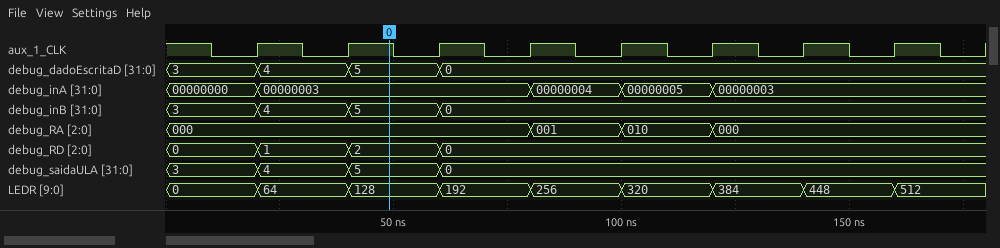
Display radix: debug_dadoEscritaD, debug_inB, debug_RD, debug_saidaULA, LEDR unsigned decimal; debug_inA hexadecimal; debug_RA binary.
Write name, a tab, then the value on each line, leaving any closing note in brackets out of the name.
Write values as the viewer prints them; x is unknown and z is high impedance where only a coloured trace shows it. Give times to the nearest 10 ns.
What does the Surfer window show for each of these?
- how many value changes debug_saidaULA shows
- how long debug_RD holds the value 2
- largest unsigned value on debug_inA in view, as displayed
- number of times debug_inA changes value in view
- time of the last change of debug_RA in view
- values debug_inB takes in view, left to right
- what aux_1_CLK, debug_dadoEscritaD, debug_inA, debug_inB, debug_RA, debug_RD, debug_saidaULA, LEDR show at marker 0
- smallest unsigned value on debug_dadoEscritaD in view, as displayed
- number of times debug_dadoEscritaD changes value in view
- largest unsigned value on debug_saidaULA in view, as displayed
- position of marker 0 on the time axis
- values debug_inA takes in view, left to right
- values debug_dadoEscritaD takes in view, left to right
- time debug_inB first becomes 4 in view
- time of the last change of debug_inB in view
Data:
how many value changes debug_saidaULA shows	3
how long debug_RD holds the value 2	20 ns
largest unsigned value on debug_inA in view, as displayed	00000005
number of times debug_inA changes value in view	4
time of the last change of debug_RA in view	120 ns
values debug_inB takes in view, left to right	3, 4, 5, 0
what aux_1_CLK, debug_dadoEscritaD, debug_inA, debug_inB, debug_RA, debug_RD, debug_saidaULA, LEDR show at marker 0	aux_1_CLK=1, debug_dadoEscritaD=5, debug_inA=00000003, debug_inB=5, debug_RA=000, debug_RD=2, debug_saidaULA=5, LEDR=128
smallest unsigned value on debug_dadoEscritaD in view, as displayed	0
number of times debug_dadoEscritaD changes value in view	3
largest unsigned value on debug_saidaULA in view, as displayed	5
position of marker 0 on the time axis	50 ns
values debug_inA takes in view, left to right	00000000, 00000003, 00000004, 00000005, 00000003
values debug_dadoEscritaD takes in view, left to right	3, 4, 5, 0
time debug_inB first becomes 4 in view	20 ns
time of the last change of debug_inB in view	60 ns
